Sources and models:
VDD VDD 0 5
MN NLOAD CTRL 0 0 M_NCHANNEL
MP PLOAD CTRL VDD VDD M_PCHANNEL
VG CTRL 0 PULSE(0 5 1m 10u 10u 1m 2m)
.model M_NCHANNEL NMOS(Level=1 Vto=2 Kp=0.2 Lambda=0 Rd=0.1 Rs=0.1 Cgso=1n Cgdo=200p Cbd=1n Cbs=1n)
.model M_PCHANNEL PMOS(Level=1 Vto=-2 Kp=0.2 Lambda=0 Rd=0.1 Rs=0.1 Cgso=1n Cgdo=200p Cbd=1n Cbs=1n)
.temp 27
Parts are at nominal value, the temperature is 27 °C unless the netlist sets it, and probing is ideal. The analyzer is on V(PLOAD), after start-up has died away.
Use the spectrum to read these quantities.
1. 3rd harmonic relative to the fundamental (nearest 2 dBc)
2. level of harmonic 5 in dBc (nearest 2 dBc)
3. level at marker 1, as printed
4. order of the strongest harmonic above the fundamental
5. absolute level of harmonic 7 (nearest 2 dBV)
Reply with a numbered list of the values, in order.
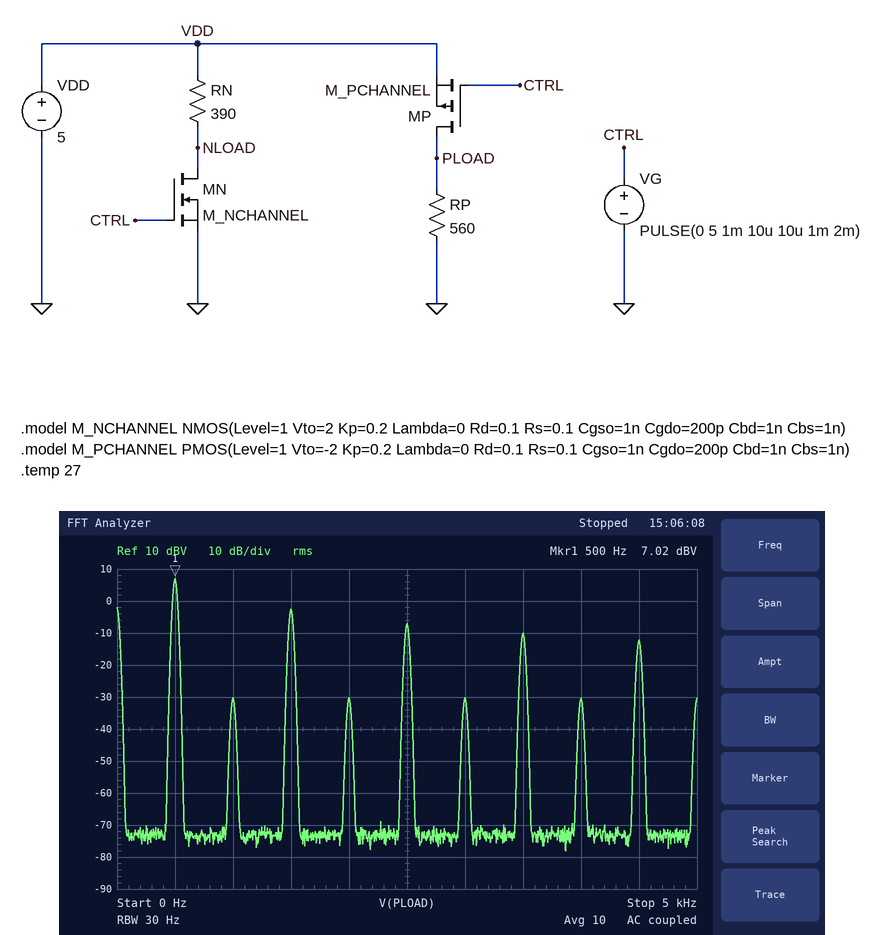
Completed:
1. -10 dBc
2. -14 dBc
3. 7.02 dBV
4. 3
5. -10 dBV
